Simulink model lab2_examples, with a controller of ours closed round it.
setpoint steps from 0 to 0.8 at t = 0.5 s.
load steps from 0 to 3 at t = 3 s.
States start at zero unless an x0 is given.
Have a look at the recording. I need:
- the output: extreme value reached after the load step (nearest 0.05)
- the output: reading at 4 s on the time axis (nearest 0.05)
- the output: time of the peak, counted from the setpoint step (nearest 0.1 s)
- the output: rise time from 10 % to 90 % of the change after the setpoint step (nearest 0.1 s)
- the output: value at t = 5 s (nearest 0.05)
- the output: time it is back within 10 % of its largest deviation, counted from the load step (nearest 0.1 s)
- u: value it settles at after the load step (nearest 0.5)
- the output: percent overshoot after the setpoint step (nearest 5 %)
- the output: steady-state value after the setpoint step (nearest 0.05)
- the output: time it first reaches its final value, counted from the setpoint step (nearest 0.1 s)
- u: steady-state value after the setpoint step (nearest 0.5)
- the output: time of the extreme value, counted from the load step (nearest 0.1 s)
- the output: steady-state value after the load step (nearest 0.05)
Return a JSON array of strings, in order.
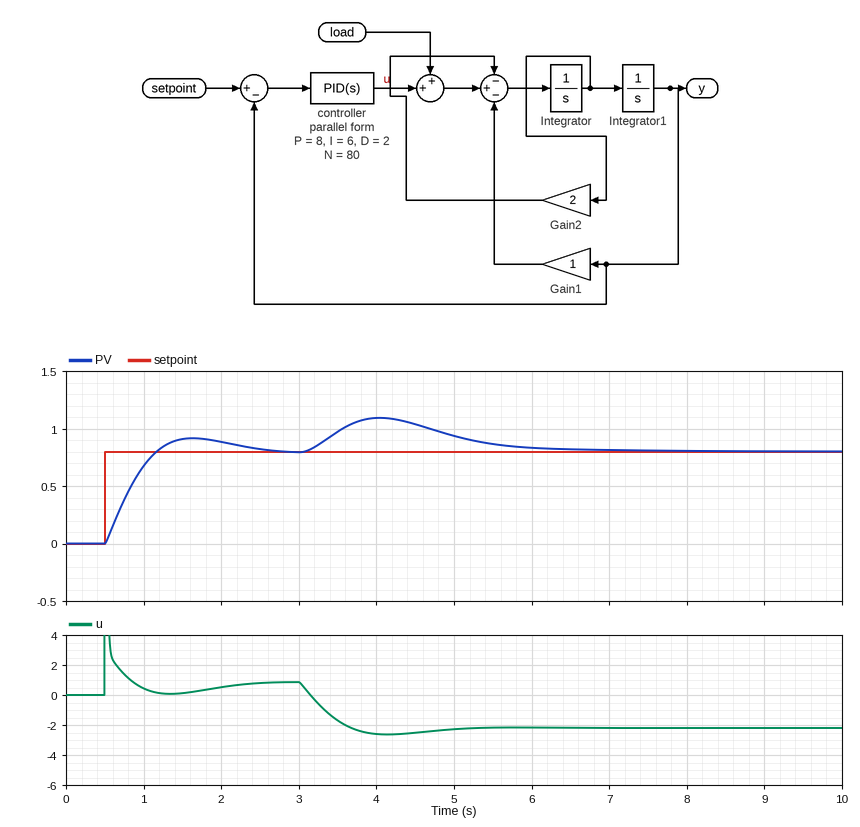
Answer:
["1.10", "1.10", "1.1 s", "0.5 s", "0.95", "3.1 s", "-2.0", "15 %", "0.80", "0.7 s", "1.0", "1.0 s", "0.80"]
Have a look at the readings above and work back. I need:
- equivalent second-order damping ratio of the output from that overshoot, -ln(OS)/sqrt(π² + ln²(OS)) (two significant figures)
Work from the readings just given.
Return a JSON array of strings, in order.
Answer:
["0.52"]
